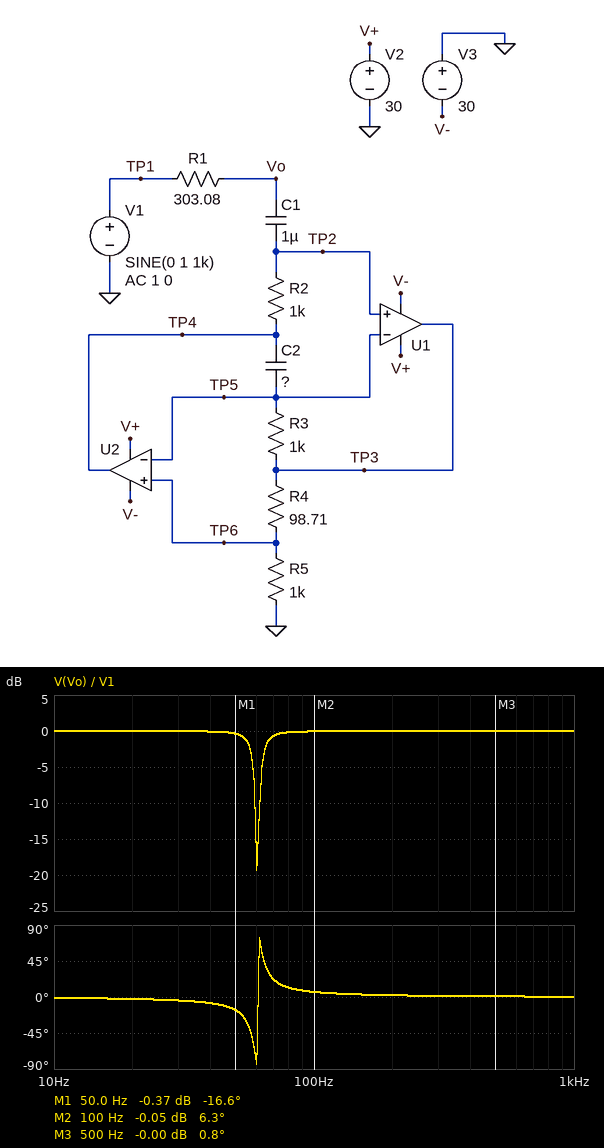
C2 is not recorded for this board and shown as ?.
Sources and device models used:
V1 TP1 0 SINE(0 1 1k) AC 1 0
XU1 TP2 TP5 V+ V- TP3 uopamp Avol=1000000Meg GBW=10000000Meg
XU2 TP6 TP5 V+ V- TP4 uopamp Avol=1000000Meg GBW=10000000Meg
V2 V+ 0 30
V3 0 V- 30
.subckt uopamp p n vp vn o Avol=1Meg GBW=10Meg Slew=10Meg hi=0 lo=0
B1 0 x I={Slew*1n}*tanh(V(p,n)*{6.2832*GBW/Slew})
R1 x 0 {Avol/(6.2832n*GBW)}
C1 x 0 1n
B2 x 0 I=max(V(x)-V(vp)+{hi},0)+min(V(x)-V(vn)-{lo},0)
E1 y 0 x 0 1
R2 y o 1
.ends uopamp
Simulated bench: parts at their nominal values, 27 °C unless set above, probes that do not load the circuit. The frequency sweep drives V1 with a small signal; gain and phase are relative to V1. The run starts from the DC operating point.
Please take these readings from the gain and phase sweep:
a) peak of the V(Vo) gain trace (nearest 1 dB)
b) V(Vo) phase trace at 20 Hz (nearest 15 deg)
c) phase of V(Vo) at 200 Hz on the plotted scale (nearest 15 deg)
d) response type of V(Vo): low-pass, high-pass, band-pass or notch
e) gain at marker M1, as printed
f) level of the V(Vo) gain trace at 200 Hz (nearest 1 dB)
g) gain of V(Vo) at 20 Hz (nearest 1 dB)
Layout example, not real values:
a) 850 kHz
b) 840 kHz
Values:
a) 0 dB
b) 0 deg
c) 0 deg
d) notch
e) -0.37 dB
f) 0 dB
g) 0 dB
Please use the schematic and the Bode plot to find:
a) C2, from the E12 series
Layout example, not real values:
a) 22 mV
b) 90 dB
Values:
a) 680 nF
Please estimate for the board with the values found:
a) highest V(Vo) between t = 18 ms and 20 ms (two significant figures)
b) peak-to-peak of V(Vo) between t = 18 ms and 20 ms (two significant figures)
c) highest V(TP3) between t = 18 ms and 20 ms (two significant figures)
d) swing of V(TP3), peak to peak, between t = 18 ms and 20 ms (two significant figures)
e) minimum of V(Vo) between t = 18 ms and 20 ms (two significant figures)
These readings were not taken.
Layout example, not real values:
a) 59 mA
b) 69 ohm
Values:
a) 1.0 V
b) 2.0 V
c) 1.1 V
d) 2.2 V
e) -1.0 V
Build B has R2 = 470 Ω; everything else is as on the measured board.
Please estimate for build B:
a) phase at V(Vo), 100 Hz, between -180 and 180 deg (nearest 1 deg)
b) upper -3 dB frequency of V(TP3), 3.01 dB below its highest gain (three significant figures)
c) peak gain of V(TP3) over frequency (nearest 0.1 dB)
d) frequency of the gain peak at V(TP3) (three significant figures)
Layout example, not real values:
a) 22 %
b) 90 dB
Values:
a) 34 deg
b) 97.8 Hz
c) 16.3 dB
d) 89.1 Hz
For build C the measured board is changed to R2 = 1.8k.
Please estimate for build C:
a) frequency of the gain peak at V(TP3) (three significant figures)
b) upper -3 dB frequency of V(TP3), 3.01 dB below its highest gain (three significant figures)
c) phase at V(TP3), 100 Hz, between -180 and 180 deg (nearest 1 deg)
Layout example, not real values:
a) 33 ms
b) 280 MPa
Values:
a) 45.3 Hz
b) 47.4 Hz
c) 3 deg
